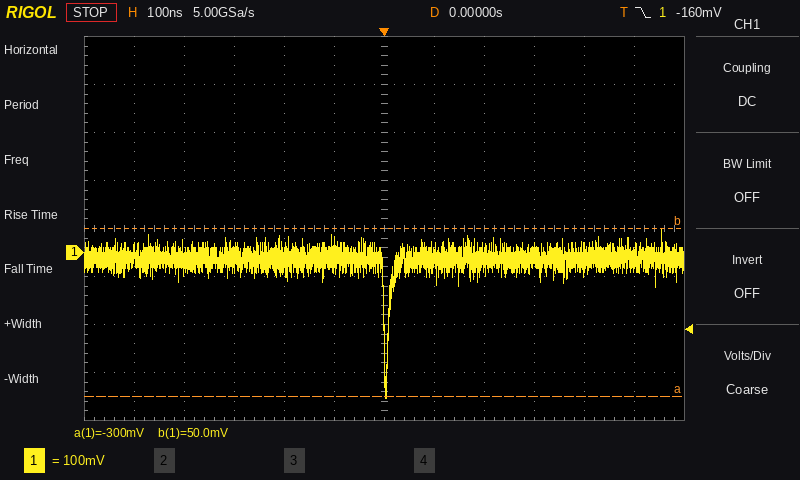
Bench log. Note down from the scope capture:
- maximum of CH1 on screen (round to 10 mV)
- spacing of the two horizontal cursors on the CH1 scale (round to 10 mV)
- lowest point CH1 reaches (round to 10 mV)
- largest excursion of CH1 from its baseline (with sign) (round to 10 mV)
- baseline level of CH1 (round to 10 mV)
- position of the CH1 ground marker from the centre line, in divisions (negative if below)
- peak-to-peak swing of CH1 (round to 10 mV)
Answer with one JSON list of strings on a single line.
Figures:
["50 mV", "350 mV", "-300 mV", "-290 mV", "-10 mV", "-0.5 div", "350 mV"]
